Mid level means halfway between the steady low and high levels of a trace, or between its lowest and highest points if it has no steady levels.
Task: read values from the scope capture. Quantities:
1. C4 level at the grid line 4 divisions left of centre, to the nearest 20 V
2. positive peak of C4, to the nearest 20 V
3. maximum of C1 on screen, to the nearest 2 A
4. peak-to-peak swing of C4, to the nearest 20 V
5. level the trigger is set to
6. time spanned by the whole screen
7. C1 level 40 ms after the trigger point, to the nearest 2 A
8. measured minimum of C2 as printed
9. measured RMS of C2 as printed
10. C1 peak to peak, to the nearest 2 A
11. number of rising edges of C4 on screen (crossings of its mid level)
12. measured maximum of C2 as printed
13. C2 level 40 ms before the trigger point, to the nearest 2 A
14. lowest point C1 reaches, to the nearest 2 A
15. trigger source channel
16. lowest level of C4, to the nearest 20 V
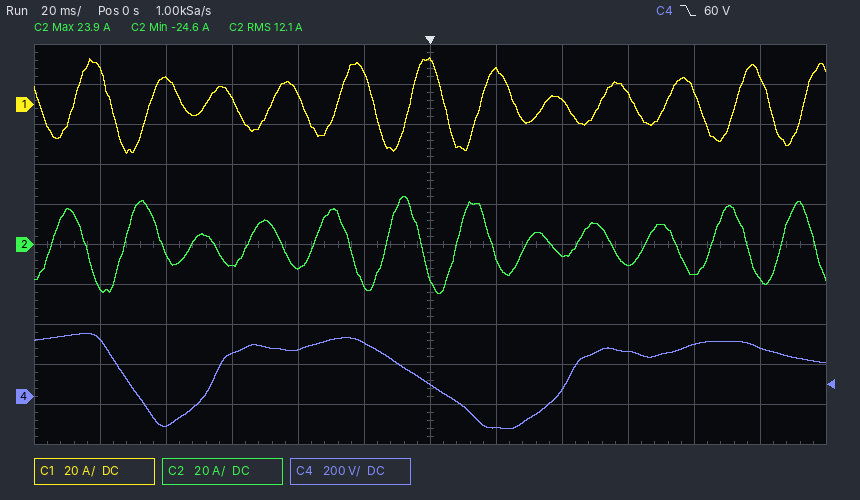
-140 V
320 V
24 A
480 V
60 V
240 ms
2 A
-24.6 A
12.1 A
48 A
2
23.9 A
-12 A
-24 A
C4
-160 V
